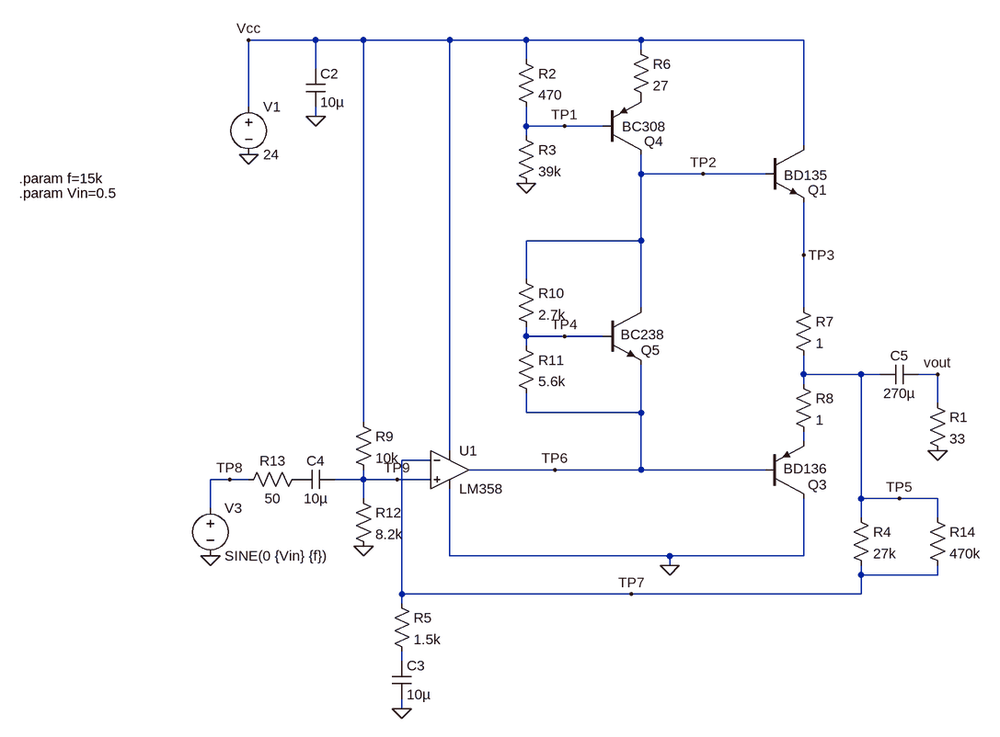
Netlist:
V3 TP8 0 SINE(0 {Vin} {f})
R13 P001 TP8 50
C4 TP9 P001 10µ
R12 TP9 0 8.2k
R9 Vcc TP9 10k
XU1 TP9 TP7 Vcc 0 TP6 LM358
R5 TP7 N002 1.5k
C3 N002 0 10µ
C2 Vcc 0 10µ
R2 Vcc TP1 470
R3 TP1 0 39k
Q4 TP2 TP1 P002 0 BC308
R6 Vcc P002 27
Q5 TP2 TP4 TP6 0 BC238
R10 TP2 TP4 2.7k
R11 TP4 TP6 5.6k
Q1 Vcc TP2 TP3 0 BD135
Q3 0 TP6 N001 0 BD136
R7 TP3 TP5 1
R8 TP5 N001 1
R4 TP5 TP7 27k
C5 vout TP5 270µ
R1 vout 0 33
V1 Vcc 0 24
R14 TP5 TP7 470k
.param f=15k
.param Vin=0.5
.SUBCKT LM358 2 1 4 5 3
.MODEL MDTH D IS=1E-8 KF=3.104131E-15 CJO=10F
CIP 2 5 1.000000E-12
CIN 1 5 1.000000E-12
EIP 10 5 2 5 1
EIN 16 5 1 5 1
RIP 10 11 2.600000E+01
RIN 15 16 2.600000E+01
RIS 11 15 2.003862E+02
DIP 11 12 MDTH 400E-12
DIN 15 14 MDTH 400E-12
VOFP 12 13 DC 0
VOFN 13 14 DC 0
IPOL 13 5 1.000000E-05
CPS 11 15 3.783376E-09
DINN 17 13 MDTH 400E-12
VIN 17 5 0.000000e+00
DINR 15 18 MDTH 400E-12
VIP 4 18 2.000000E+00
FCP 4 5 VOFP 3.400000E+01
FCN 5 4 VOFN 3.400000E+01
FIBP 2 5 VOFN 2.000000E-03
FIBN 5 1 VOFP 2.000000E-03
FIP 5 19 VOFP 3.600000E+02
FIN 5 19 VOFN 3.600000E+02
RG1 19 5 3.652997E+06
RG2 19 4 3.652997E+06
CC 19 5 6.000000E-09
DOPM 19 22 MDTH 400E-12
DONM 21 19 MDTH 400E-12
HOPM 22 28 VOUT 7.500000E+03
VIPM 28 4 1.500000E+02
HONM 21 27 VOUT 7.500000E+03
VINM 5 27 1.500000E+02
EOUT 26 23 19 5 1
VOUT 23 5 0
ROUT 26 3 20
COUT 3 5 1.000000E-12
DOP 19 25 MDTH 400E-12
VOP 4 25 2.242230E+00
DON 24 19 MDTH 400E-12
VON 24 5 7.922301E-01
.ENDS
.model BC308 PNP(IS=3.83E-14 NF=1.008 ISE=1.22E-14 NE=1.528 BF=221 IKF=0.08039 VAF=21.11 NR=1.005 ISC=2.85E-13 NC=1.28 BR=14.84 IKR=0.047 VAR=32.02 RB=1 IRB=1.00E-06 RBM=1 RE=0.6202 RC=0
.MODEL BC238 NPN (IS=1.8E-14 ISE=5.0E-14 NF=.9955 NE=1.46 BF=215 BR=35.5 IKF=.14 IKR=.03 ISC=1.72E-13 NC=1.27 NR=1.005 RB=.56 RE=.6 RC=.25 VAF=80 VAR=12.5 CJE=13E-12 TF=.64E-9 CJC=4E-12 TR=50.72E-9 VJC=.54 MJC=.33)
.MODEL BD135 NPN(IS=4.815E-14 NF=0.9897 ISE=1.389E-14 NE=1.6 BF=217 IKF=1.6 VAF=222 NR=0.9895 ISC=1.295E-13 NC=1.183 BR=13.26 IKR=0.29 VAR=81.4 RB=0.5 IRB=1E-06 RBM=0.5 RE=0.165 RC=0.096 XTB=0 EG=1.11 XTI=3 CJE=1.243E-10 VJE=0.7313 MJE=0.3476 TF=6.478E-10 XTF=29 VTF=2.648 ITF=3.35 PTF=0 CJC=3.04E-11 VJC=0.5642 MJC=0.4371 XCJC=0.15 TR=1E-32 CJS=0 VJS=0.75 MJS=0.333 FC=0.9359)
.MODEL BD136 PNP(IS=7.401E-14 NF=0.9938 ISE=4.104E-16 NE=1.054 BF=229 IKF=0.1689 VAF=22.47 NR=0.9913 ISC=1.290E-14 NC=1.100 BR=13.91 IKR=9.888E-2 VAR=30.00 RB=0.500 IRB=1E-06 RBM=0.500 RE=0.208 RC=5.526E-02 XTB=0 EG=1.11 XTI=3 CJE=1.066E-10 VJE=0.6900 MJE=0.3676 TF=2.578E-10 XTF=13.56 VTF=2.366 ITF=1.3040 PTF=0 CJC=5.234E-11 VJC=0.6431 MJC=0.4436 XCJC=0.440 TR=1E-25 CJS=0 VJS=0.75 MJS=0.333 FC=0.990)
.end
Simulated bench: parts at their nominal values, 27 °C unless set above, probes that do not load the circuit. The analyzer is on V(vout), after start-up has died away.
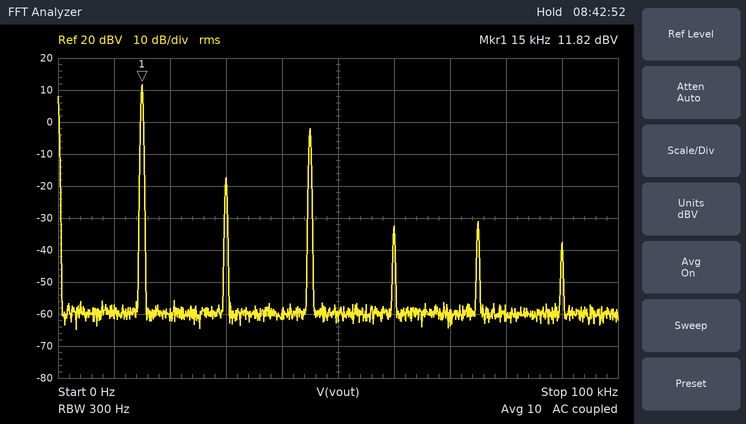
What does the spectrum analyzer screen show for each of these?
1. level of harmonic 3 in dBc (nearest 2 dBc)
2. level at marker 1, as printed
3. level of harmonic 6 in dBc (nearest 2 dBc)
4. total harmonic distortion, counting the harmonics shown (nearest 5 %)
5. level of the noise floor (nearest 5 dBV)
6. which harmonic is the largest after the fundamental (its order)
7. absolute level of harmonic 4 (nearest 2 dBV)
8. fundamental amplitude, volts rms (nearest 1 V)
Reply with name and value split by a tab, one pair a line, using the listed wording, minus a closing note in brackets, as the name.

level of harmonic 3 in dBc	-14 dBc
level at marker 1, as printed	11.82 dBV
level of harmonic 6 in dBc	-50 dBc
total harmonic distortion, counting the harmonics shown	20 %
level of the noise floor	-60 dBV
which harmonic is the largest after the fundamental	3
absolute level of harmonic 4	-32 dBV
fundamental amplitude, volts rms	4 V
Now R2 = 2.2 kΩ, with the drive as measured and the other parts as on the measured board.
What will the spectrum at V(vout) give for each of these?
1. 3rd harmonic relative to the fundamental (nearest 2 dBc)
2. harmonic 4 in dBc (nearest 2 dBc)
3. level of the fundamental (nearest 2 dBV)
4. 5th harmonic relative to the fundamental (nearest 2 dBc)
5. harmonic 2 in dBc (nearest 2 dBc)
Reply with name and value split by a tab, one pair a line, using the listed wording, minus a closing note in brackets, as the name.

3rd harmonic relative to the fundamental	-22 dBc
harmonic 4 in dBc	-42 dBc
level of the fundamental	14 dBV
5th harmonic relative to the fundamental	-38 dBc
harmonic 2 in dBc	-40 dBc
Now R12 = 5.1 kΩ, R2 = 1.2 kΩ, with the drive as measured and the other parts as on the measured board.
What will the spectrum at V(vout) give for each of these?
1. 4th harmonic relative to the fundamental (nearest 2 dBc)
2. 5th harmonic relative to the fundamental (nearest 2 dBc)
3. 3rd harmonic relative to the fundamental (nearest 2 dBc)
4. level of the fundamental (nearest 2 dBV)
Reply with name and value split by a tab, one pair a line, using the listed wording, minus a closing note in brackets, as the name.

4th harmonic relative to the fundamental	-38 dBc
5th harmonic relative to the fundamental	-42 dBc
3rd harmonic relative to the fundamental	-22 dBc
level of the fundamental	14 dBV
